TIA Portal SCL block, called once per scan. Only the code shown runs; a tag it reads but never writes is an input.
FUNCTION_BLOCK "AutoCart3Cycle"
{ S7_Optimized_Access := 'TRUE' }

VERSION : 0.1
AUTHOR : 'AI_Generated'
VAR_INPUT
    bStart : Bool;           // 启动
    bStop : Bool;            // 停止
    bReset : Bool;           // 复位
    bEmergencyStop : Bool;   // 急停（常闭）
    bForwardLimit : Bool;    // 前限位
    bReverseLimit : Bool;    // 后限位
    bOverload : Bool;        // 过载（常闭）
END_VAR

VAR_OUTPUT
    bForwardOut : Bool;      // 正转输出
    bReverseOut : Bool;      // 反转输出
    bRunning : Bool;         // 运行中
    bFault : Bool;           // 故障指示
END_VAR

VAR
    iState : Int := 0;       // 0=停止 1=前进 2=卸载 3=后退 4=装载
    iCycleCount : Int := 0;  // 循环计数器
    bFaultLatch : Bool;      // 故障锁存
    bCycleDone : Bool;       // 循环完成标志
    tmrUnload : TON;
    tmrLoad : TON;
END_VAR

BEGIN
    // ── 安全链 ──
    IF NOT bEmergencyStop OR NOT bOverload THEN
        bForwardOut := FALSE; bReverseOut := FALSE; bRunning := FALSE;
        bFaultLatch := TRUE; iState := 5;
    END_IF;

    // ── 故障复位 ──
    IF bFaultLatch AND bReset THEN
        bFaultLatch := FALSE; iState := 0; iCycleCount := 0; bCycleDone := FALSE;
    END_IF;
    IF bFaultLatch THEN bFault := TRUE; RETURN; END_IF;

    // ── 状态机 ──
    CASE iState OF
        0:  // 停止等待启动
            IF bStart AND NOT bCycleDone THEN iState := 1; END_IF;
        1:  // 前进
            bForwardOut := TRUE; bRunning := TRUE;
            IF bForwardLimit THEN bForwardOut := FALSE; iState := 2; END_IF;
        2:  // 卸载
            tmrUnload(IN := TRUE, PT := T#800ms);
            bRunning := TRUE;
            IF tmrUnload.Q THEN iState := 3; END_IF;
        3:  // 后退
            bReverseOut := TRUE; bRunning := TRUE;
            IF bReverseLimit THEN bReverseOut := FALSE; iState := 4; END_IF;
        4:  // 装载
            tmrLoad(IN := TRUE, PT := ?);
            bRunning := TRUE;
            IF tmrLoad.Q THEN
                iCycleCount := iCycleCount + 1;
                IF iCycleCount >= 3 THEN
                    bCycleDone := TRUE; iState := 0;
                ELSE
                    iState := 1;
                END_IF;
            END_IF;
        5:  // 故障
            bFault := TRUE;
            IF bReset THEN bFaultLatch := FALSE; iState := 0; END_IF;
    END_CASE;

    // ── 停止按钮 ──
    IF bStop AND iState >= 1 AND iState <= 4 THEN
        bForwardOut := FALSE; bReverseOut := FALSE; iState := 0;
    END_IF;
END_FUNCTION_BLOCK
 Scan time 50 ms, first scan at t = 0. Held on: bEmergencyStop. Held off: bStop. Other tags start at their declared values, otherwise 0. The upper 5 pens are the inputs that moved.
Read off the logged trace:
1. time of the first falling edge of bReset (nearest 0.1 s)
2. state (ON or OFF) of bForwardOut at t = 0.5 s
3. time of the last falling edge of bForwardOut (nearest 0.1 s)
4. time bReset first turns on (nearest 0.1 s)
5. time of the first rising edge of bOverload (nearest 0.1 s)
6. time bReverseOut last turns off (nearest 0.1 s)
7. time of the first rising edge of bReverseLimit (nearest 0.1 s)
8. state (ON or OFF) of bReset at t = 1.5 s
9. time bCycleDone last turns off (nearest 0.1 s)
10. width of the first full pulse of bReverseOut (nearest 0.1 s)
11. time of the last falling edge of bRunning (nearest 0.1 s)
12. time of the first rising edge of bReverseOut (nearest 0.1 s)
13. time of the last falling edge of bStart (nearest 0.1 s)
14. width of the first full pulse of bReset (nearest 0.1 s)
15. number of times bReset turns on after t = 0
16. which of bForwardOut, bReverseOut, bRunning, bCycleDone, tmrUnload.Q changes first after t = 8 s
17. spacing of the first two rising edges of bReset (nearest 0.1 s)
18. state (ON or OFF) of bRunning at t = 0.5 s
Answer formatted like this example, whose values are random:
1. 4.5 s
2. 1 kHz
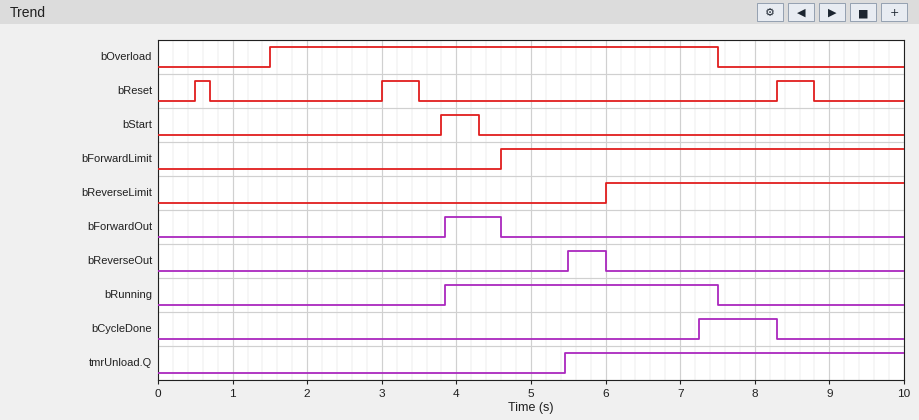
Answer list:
1. 0.7 s
2. OFF
3. 4.6 s
4. 0.5 s
5. 1.5 s
6. 6.0 s
7. 6.0 s
8. OFF
9. 8.3 s
10. 0.5 s
11. 7.5 s
12. 5.5 s
13. 4.3 s
14. 0.2 s
15. 3
16. bCycleDone
17. 2.5 s
18. OFF
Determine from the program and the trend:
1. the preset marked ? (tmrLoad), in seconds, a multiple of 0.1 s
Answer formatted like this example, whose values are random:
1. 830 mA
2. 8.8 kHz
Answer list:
1. 0.8 s
